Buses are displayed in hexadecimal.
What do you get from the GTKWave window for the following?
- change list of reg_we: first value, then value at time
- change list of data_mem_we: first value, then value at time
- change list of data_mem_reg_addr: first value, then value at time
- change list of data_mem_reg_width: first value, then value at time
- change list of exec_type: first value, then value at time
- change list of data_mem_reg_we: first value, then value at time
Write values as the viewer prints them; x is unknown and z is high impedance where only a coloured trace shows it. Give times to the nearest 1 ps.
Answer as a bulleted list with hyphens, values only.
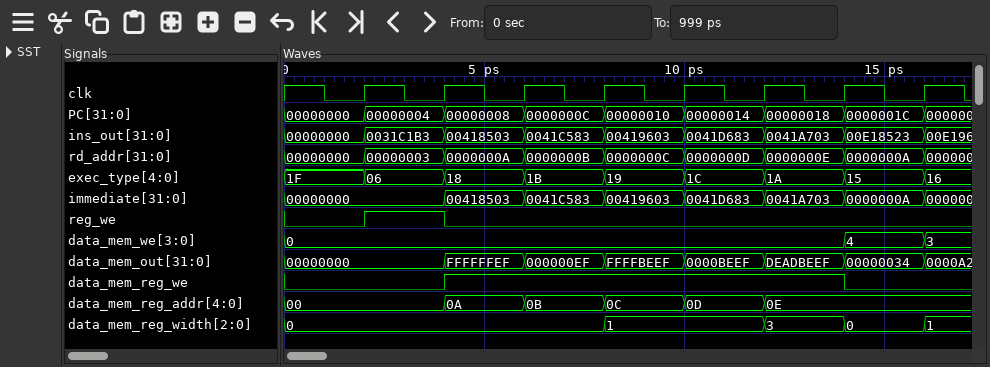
- 0, 1 at 2 ps, 0 at 4 ps
- 0, 4 at 14 ps, 3 at 16 ps
- 00, 0A at 4 ps, 0B at 6 ps, 0C at 8 ps, 0D at 10 ps, 0E at 12 ps
- 0, 1 at 8 ps, 3 at 12 ps, 0 at 14 ps, 1 at 16 ps
- 1F, 06 at 2 ps, 18 at 4 ps, 1B at 6 ps, 19 at 8 ps, 1C at 10 ps, 1A at 12 ps, 15 at 14 ps, 16 at 16 ps
- 0, 1 at 4 ps, 0 at 14 ps
